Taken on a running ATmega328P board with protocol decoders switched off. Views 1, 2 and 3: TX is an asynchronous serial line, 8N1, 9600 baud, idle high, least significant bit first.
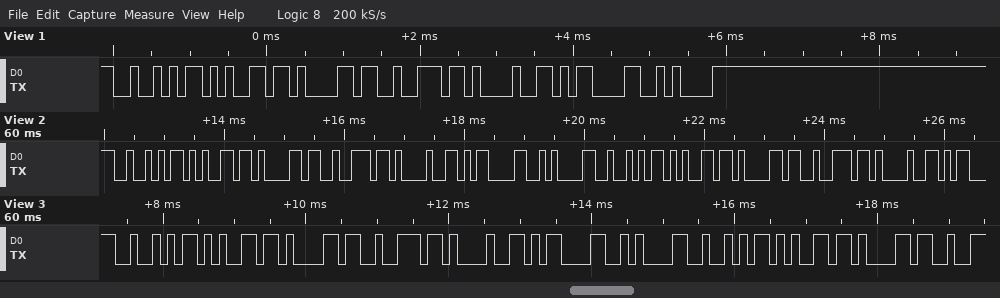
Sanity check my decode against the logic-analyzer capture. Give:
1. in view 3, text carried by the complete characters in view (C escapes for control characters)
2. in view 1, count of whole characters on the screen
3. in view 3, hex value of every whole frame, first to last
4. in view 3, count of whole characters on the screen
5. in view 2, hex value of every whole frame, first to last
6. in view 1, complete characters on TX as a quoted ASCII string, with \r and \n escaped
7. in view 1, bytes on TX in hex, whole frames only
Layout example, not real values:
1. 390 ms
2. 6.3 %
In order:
1. "Rear!\r\nRea"
2. 7
3. 52 65 61 72 21 0D 0A 52 65 61
4. 10
5. 0x52 0x65 0x61 0x72 0x21 0x0D 0x0A 0x52 0x65 0x61 0x72 0x21
6. "Rear!\r\n"
7. 52 65 61 72 21 0D 0A
